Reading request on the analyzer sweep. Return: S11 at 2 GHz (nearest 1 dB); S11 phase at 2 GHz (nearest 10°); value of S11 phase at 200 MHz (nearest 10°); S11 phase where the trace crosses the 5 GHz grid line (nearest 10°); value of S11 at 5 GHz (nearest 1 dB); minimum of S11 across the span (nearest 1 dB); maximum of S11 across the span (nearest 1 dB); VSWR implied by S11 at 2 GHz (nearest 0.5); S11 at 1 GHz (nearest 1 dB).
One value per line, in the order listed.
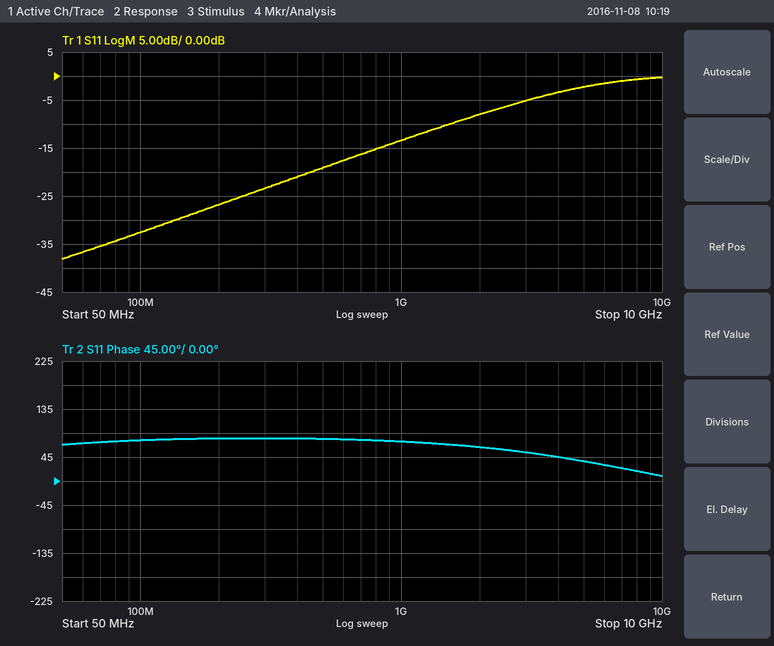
-8 dB
60°
80°
40°
-2 dB
-38 dB
0 dB
2.5
-13 dB
